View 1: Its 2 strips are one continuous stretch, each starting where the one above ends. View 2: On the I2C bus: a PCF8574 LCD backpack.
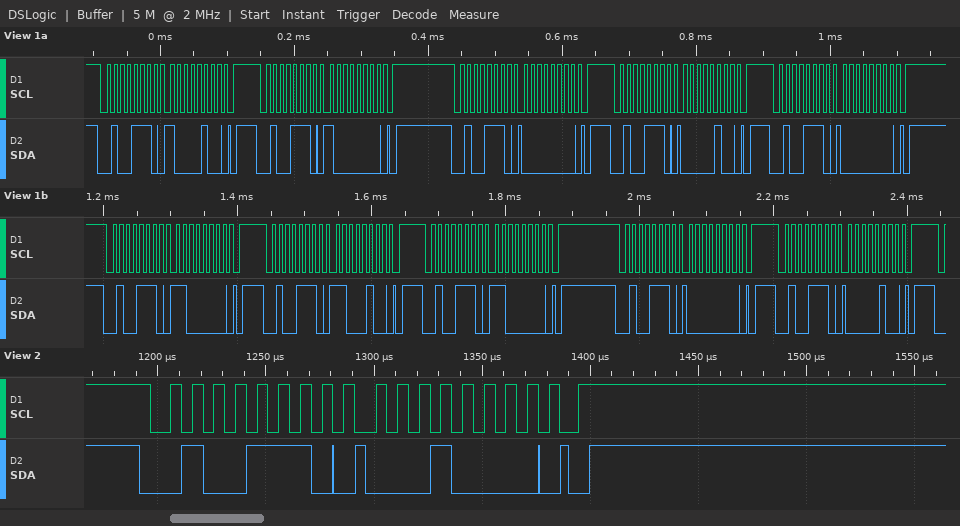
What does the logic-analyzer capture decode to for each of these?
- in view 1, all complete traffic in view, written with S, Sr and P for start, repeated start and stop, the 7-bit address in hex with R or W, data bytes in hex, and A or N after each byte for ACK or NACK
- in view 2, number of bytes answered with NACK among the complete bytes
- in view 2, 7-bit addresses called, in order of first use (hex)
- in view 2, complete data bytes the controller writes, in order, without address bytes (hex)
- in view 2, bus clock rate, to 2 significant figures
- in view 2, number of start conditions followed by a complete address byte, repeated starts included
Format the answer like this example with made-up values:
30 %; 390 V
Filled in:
S 27W A 84 A P S 27W A 80 A P S 27W A 00 A P S 27W A 04 A P S 27W A 00 A P S 27W A C0 A P S 27W A C4 A P S 27W A C0 A P S 27W A 00 A P S 27W A 04 A P; 0; 0x27; 10; 100 kHz; 1
